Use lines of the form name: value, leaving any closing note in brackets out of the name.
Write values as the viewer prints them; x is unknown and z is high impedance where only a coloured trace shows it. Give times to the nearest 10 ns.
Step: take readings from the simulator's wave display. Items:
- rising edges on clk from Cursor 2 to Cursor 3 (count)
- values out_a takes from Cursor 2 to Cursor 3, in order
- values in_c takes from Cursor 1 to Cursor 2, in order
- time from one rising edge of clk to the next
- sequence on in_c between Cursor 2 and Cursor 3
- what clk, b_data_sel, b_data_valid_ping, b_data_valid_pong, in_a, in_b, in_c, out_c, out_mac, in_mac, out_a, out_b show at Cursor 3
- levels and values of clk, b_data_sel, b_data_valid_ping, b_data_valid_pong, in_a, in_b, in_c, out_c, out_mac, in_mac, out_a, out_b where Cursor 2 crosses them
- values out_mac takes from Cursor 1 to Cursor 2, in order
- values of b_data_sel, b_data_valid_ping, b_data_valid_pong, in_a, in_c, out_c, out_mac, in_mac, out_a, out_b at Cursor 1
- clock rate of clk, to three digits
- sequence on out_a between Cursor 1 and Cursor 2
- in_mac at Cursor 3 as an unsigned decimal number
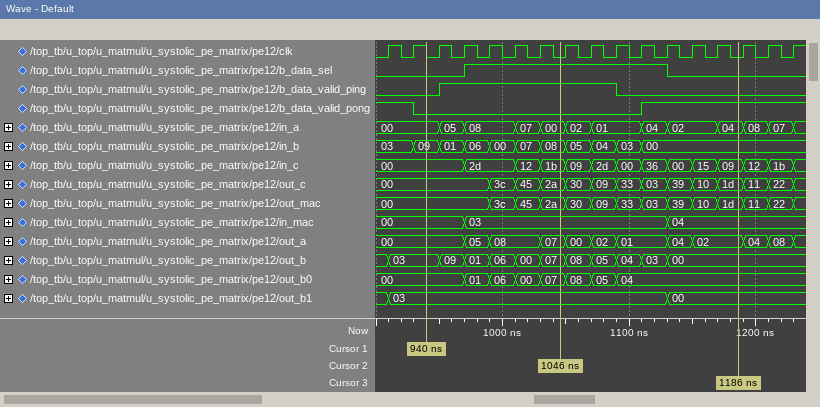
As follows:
rising edges on clk from Cursor 2 to Cursor 3: 7
values out_a takes from Cursor 2 to Cursor 3, in order: 07, 00, 02, 01, 04, 02
values in_c takes from Cursor 1 to Cursor 2, in order: 00, 2d, 12, 1b
time from one rising edge of clk to the next: 20 ns
sequence on in_c between Cursor 2 and Cursor 3: 1b, 09, 2d, 00, 36, 00, 15, 09
what clk, b_data_sel, b_data_valid_ping, b_data_valid_pong, in_a, in_b, in_c, out_c, out_mac, in_mac, out_a, out_b show at Cursor 3: clk=0, b_data_sel=0, b_data_valid_ping=0, b_data_valid_pong=1, in_a=04, in_b=00, in_c=09, out_c=1d, out_mac=1d, in_mac=04, out_a=02, out_b=00
levels and values of clk, b_data_sel, b_data_valid_ping, b_data_valid_pong, in_a, in_b, in_c, out_c, out_mac, in_mac, out_a, out_b where Cursor 2 crosses them: clk=0, b_data_sel=1, b_data_valid_ping=1, b_data_valid_pong=0, in_a=00, in_b=08, in_c=1b, out_c=2a, out_mac=2a, in_mac=03, out_a=07, out_b=07
values out_mac takes from Cursor 1 to Cursor 2, in order: 00, 3c, 45, 2a
values of b_data_sel, b_data_valid_ping, b_data_valid_pong, in_a, in_c, out_c, out_mac, in_mac, out_a, out_b at Cursor 1: b_data_sel=0, b_data_valid_ping=0, b_data_valid_pong=0, in_a=00, in_c=00, out_c=00, out_mac=00, in_mac=00, out_a=00, out_b=03
clock rate of clk, to three digits: 50.0 MHz
sequence on out_a between Cursor 1 and Cursor 2: 00, 05, 08, 07
in_mac at Cursor 3 as an unsigned decimal number: 4
